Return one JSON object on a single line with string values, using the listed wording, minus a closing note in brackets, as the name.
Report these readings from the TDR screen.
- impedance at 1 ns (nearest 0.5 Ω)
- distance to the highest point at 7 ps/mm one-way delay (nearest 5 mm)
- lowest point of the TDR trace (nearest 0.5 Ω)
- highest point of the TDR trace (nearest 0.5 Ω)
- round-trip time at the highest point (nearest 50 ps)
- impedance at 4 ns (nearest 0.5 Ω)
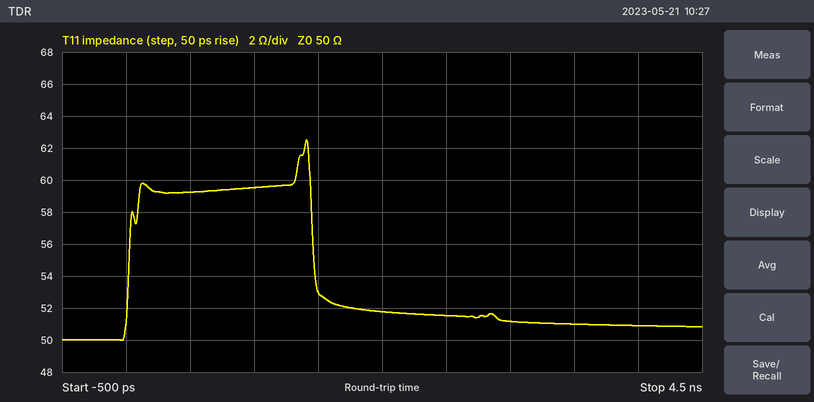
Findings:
{"impedance at 1 ns": "59.5 Ω", "distance to the highest point at 7 ps/mm one-way delay": "100 mm", "lowest point of the TDR trace": "50.0 Ω", "highest point of the TDR trace": "62.5 Ω", "round-trip time at the highest point": "1.40 ns", "impedance at 4 ns": "51.0 Ω"}
